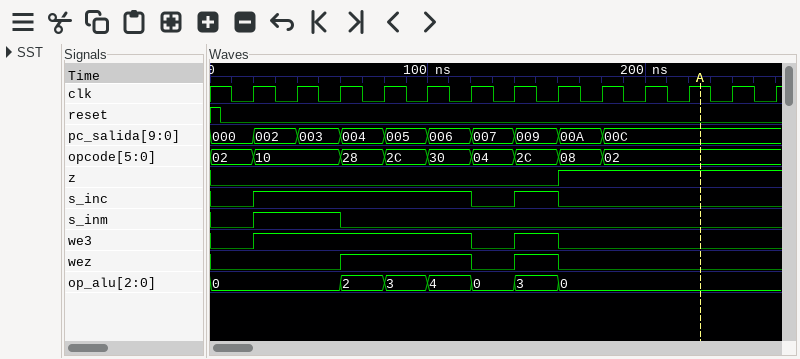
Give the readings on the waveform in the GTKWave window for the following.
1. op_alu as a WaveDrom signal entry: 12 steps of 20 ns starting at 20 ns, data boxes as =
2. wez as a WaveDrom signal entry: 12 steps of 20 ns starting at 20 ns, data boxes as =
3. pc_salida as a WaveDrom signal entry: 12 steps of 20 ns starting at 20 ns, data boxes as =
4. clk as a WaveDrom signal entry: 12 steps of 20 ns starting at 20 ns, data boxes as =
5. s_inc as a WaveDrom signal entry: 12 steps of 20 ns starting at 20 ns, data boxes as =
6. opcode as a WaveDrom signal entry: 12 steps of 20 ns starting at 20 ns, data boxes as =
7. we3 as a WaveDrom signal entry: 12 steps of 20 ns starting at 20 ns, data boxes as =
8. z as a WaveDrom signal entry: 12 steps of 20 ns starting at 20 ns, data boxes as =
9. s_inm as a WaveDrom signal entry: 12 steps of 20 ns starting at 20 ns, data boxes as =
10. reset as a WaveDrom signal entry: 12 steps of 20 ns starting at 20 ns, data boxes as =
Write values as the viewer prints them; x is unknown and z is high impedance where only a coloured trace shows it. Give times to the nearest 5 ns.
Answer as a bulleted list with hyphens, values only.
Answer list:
- {name: 'op_alu', wave: '=.======....', data: '0 2 3 4 0 3 0'}
- {name: 'wez', wave: '0.1..010....'}
- {name: 'pc_salida', wave: '=========...', data: '002 003 004 005 006 007 009 00A 00C'}
- {name: 'clk', wave: 'p...........'}
- {name: 's_inc', wave: '1....010....'}
- {name: 'opcode', wave: '=.=======...', data: '10 28 2C 30 04 2C 08 02'}
- {name: 'we3', wave: '1....010....'}
- {name: 'z', wave: '0......1....'}
- {name: 's_inm', wave: '1.0.........'}
- {name: 'reset', wave: '0...........'}
